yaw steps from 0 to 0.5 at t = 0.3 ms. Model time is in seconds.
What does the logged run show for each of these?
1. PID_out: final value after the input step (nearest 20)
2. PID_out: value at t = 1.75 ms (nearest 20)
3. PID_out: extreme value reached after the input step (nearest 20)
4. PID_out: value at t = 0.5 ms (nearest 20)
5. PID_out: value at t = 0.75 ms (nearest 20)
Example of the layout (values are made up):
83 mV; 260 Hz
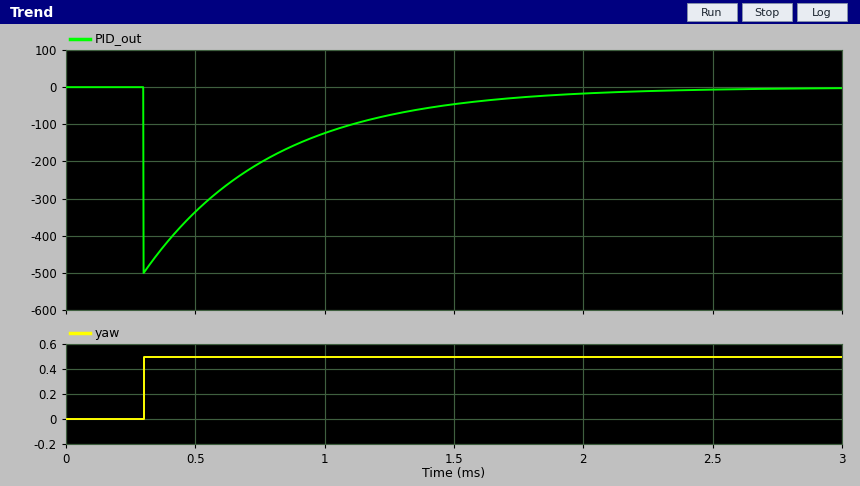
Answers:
0; -20; -500; -340; -200
